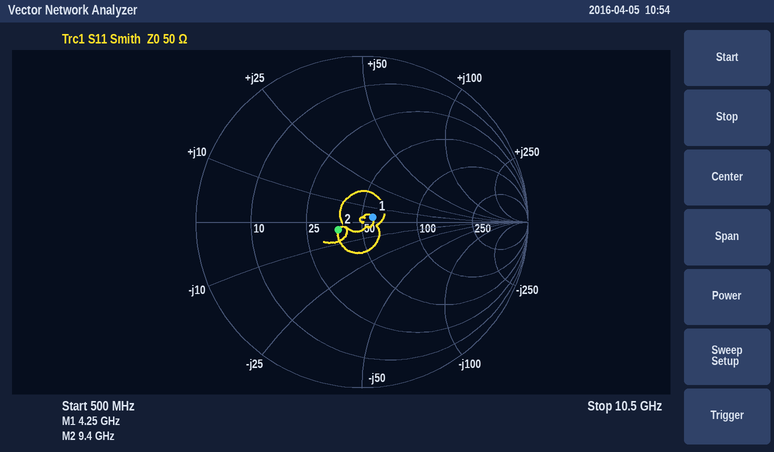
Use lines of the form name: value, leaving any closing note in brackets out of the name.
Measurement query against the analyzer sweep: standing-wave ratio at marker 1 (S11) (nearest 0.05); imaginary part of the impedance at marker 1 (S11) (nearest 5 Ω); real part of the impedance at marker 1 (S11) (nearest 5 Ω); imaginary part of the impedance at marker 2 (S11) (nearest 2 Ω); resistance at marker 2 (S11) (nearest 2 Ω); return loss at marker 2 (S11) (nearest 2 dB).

standing-wave ratio at marker 1 (S11): 1.15
imaginary part of the impedance at marker 1 (S11): +5 Ω
real part of the impedance at marker 1 (S11): 55 Ω
imaginary part of the impedance at marker 2 (S11): -4 Ω
resistance at marker 2 (S11): 38 Ω
return loss at marker 2 (S11): 16 dB
